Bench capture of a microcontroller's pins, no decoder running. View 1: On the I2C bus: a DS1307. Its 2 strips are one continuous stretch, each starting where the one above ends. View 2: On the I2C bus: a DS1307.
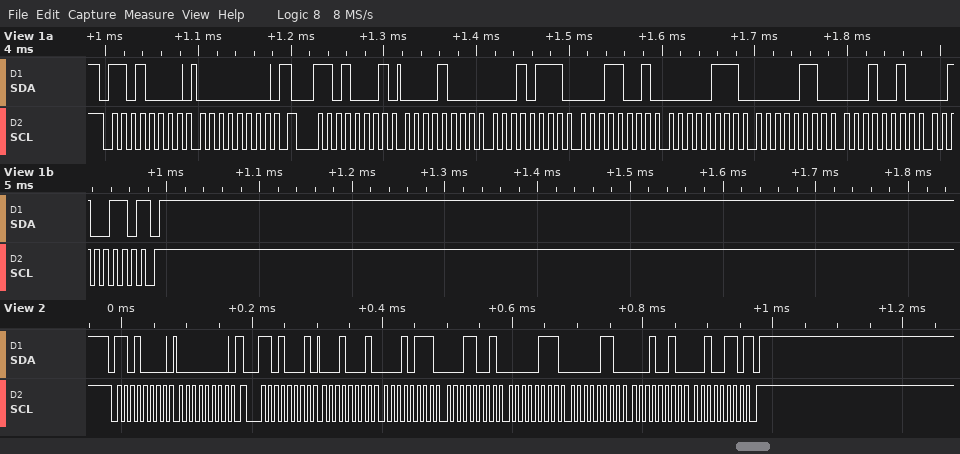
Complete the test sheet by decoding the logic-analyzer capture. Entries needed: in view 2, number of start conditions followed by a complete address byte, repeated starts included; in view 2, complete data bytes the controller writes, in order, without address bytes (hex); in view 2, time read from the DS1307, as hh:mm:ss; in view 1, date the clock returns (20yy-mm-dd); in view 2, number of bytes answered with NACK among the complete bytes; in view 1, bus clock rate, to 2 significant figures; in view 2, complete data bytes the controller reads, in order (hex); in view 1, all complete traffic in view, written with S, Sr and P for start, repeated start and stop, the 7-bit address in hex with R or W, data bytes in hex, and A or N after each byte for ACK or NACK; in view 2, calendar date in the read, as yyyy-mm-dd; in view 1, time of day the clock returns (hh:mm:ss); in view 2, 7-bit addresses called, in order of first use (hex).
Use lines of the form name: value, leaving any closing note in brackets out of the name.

in view 2, number of start conditions followed by a complete address byte, repeated starts included: 2
in view 2, complete data bytes the controller writes, in order, without address bytes: 00
in view 2, time read from the DS1307, as hh:mm:ss: 19:17:11
in view 1, date the clock returns: 2026-12-06
in view 2, number of bytes answered with NACK among the complete bytes: 1
in view 1, bus clock rate, to 2 significant figures: 100 kHz
in view 2, complete data bytes the controller reads, in order: 11 17 19 07 06 12 26
in view 1, all complete traffic in view, written with S, Sr and P for start, repeated start and stop, the 7-bit address in hex with R or W, data bytes in hex, and A or N after each byte for ACK or NACK: S 68W A 00 A Sr 68R A 08 A 17 A 19 A 07 A 06 A 12 A 26 N P
in view 2, calendar date in the read, as yyyy-mm-dd: 2026-12-06
in view 1, time of day the clock returns: 19:17:08
in view 2, 7-bit addresses called, in order of first use: 0x68
